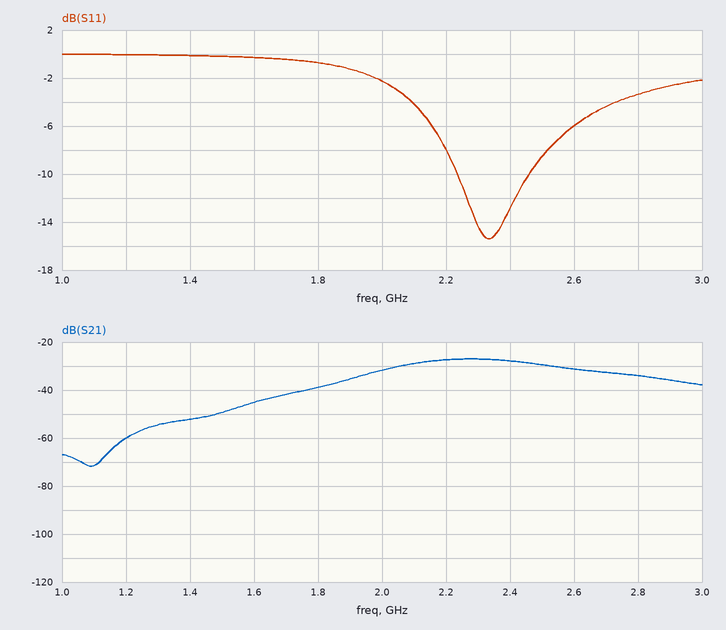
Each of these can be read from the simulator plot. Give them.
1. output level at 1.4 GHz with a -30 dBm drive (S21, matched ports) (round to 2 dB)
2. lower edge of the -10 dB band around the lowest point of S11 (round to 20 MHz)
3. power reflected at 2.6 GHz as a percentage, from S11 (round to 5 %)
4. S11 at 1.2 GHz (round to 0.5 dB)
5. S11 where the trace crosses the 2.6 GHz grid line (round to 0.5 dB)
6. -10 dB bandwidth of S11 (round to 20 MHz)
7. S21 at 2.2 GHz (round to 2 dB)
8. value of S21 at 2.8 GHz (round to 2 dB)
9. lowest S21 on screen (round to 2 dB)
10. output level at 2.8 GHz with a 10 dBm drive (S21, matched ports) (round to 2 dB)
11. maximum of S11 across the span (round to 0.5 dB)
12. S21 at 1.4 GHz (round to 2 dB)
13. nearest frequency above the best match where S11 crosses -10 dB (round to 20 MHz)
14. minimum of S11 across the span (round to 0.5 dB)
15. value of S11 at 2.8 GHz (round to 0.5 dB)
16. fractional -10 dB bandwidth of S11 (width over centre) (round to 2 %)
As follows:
-82 dBm
2.24 GHz
25 %
0.0 dB
-6.0 dB
220 MHz
-28 dB
-34 dB
-72 dB
-24 dBm
0.0 dB
-52 dB
2.46 GHz
-15.5 dB
-3.5 dB
10 %
